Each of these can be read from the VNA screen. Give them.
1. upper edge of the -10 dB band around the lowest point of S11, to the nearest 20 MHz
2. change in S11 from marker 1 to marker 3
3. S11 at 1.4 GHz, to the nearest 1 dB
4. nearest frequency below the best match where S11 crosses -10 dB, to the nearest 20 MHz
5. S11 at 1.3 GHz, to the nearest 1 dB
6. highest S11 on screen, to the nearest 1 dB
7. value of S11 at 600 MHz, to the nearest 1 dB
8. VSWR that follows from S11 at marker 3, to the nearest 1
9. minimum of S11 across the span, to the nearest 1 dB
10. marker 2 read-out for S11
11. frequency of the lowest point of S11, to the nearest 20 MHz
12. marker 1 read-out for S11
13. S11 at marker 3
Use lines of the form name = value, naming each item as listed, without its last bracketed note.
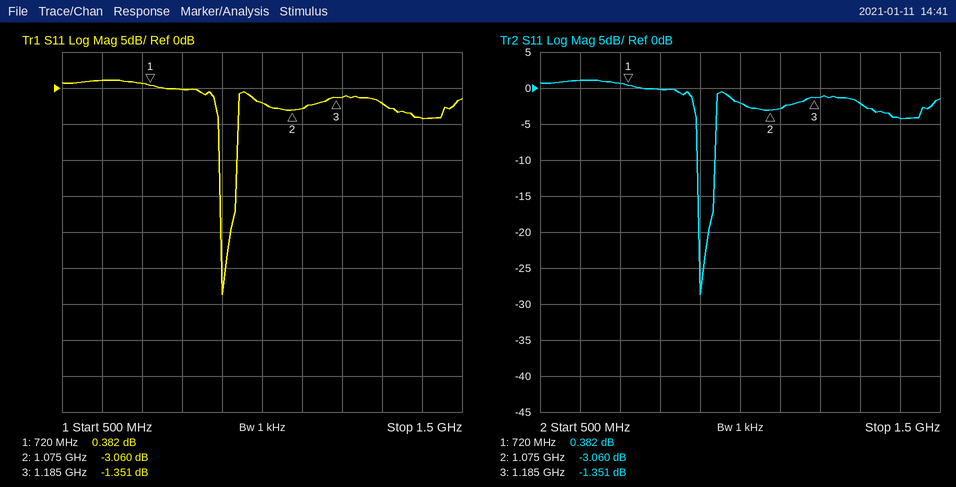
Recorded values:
upper edge of the -10 dB band around the lowest point of S11, to the nearest 20 MHz = 940 MHz
change in S11 from marker 1 to marker 3 = -1.733 dB
S11 at 1.4 GHz, to the nearest 1 dB = -4 dB
nearest frequency below the best match where S11 crosses -10 dB, to the nearest 20 MHz = 900 MHz
S11 at 1.3 GHz, to the nearest 1 dB = -2 dB
highest S11 on screen, to the nearest 1 dB = 1 dB
value of S11 at 600 MHz, to the nearest 1 dB = 1 dB
VSWR that follows from S11 at marker 3, to the nearest 1 = 13
minimum of S11 across the span, to the nearest 1 dB = -29 dB
marker 2 read-out for S11 = -3.060 dB
frequency of the lowest point of S11, to the nearest 20 MHz = 900 MHz
marker 1 read-out for S11 = 0.382 dB
S11 at marker 3 = -1.351 dB
